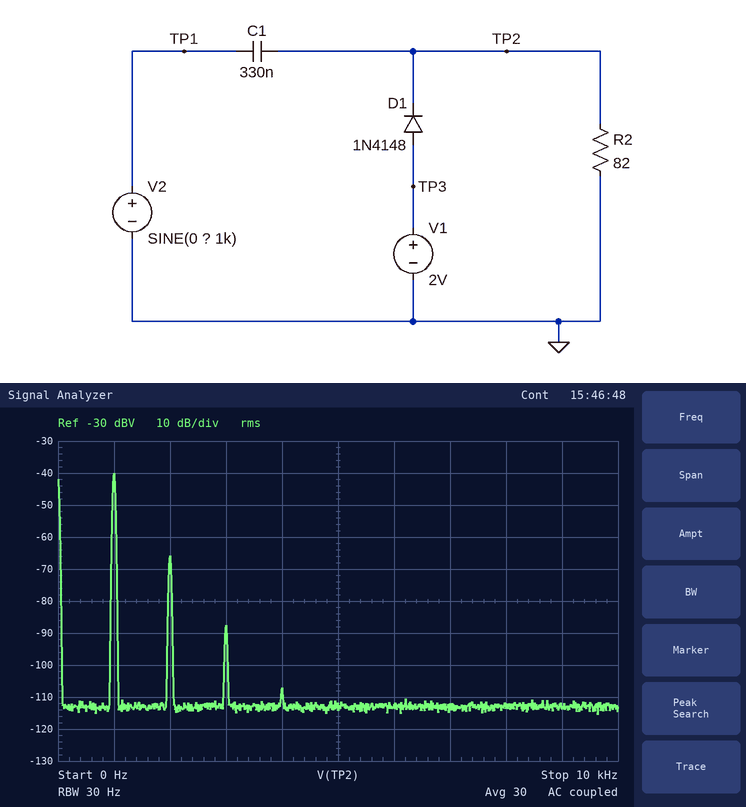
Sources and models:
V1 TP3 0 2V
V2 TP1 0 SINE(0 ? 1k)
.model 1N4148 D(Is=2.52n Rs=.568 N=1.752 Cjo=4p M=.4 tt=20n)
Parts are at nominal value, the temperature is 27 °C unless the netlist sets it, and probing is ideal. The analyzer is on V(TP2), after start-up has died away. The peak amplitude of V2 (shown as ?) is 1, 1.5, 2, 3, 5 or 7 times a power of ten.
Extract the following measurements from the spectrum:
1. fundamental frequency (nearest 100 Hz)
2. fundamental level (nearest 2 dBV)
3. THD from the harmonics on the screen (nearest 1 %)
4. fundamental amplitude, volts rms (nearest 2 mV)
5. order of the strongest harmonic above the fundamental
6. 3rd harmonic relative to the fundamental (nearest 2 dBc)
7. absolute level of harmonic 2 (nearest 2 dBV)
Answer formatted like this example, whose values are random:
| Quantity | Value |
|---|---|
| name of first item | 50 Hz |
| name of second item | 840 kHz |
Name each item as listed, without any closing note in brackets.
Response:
| Quantity | Value |
|---|---|
| fundamental frequency | 1.0 kHz |
| fundamental level | -40 dBV |
| THD from the harmonics on the screen | 5 % |
| fundamental amplitude, volts rms | 10 mV |
| order of the strongest harmonic above the fundamental | 2 |
| 3rd harmonic relative to the fundamental | -48 dBc |
| absolute level of harmonic 2 | -66 dBV |
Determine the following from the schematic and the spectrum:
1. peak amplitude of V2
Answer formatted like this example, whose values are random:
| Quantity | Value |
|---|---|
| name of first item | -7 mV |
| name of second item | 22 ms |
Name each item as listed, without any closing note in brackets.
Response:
| Quantity | Value |
|---|---|
| peak amplitude of V2 | 2 V |
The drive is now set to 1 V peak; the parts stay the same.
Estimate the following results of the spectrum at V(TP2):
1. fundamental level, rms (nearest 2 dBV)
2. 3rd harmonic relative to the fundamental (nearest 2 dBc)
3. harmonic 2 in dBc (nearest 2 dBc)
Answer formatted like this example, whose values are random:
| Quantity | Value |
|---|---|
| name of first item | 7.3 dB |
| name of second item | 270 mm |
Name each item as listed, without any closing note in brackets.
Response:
| Quantity | Value |
|---|---|
| fundamental level, rms | -46 dBV |
| 3rd harmonic relative to the fundamental | -60 dBc |
| harmonic 2 in dBc | -32 dBc |
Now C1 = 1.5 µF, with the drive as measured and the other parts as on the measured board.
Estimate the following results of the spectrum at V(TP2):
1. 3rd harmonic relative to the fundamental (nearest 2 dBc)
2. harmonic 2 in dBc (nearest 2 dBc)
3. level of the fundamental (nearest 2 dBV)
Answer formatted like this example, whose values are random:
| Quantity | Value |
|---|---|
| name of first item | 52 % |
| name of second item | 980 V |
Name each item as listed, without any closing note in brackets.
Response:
| Quantity | Value |
|---|---|
| 3rd harmonic relative to the fundamental | -14 dBc |
| harmonic 2 in dBc | -8 dBc |
| level of the fundamental | -22 dBV |
